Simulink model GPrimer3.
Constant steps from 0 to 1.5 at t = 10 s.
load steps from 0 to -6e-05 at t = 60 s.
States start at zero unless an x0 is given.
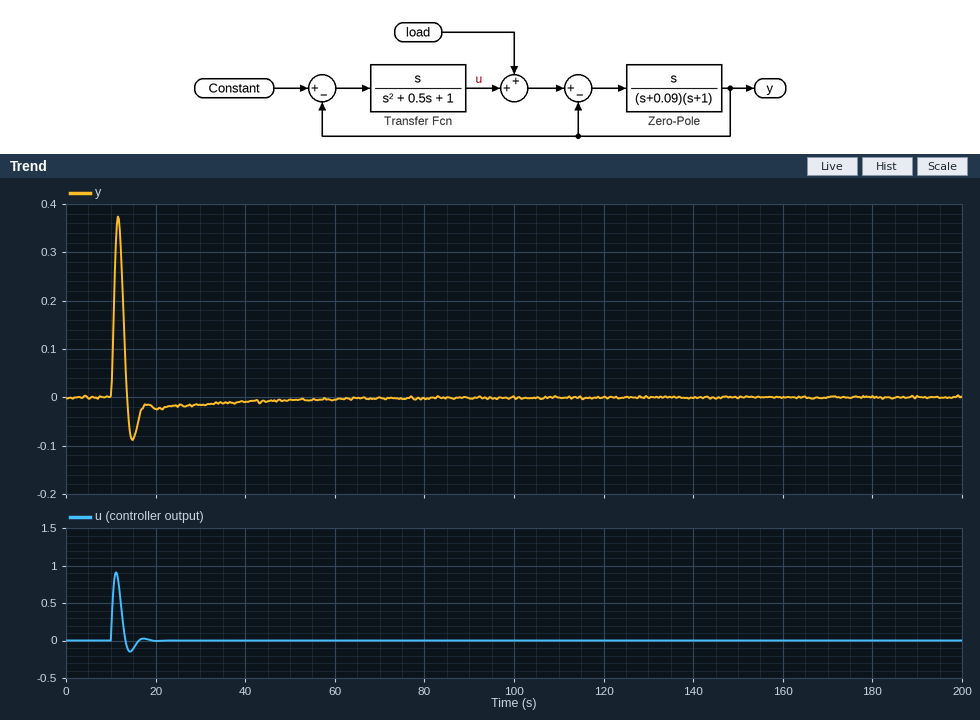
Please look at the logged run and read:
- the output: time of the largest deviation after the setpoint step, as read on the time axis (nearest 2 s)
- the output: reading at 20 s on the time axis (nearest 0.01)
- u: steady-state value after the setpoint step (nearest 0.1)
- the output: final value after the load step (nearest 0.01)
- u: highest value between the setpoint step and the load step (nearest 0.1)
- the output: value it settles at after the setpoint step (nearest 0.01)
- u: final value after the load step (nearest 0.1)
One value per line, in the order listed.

12 s
-0.02
0.0
0.00
0.9
0.00
0.0
